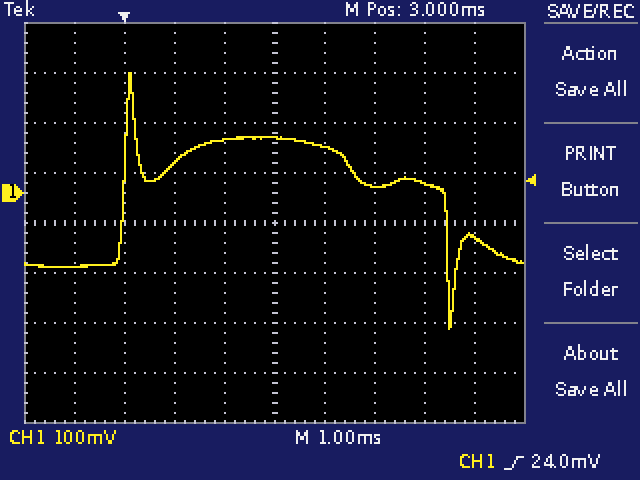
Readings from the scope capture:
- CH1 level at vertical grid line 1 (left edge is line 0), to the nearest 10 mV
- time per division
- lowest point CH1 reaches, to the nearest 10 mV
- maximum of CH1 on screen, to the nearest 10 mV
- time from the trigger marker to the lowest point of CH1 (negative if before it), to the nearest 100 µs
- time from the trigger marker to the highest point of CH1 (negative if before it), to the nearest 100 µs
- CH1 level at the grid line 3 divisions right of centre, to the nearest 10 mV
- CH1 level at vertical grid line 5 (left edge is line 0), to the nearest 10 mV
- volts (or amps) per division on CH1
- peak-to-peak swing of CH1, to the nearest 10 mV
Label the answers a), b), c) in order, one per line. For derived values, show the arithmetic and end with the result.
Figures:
a) -150 mV
b) 1 ms
c) -270 mV
d) 240 mV
e) +6.5 ms
f) +100 µs
g) 20 mV
h) 110 mV
i) 100 mV
j) 240 mV − (-270 mV) = 510 mV
